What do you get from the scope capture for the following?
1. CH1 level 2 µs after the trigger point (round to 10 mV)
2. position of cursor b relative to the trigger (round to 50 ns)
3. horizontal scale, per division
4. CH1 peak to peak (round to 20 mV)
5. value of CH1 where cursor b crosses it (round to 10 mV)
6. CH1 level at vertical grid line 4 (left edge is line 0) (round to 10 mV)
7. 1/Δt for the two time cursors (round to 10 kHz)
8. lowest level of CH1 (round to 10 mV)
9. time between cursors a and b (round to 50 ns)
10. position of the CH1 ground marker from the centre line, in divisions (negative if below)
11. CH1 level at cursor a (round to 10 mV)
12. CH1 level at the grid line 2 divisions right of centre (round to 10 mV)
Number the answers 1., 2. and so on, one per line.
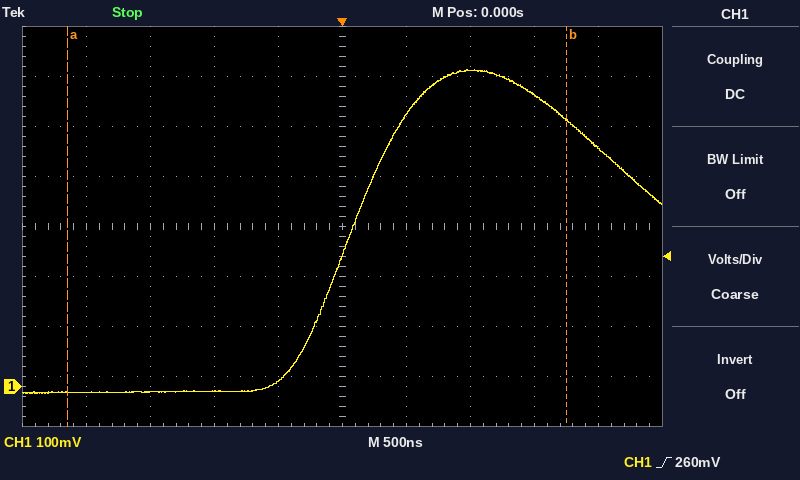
1. 480 mV
2. +1.75 µs
3. 500 ns
4. 640 mV
5. 530 mV
6. 10 mV
7. 260 kHz
8. -10 mV
9. 3.90 µs
10. -3.2 div
11. -10 mV
12. 630 mV
